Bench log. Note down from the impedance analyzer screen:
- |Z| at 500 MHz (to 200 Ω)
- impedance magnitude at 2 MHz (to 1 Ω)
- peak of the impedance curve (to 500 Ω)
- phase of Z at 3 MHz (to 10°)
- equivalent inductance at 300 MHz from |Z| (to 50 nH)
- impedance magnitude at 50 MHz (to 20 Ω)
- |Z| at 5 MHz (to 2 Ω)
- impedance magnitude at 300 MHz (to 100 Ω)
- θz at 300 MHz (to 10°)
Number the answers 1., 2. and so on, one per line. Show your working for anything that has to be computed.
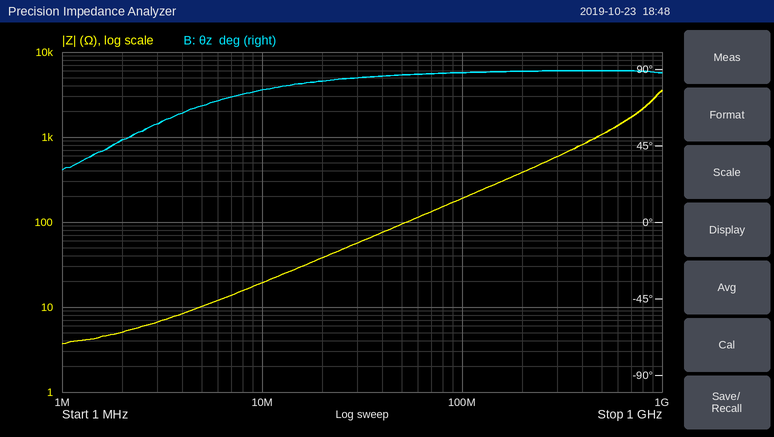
1. 1.0 kΩ
2. 5 Ω
3. 3.5 kΩ
4. 60°
5. L = 600 Ω/(2π × 300 MHz) ≈ 318 nH, so 300 nH to the nearest 50 nH
6. 100 Ω
7. 10 Ω
8. 600 Ω
9. 90°
